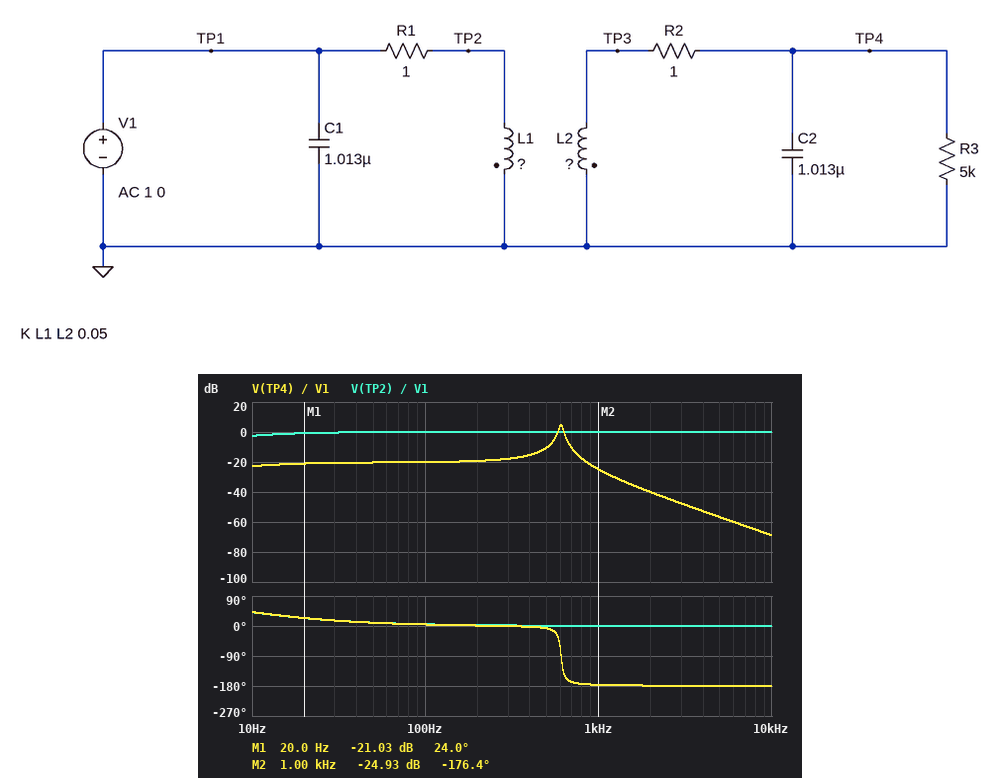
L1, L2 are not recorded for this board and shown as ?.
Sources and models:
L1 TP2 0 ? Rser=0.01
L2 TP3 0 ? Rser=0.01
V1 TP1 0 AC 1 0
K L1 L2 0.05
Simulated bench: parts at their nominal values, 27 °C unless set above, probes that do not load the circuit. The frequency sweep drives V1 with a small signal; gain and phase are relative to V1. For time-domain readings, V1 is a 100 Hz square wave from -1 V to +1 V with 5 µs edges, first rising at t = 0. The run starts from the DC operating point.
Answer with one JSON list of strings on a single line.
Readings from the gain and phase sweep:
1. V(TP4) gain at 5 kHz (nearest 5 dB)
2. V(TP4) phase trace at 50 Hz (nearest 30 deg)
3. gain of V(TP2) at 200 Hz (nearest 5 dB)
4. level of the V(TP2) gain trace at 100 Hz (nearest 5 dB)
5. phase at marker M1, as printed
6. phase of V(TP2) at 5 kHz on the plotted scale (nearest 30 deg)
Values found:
["-55 dB", "0 deg", "0 dB", "0 dB", "24.0 deg", "0 deg"]
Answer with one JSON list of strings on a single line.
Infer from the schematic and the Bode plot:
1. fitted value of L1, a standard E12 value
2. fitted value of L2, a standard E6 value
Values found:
["18 mH", "68 mH"]
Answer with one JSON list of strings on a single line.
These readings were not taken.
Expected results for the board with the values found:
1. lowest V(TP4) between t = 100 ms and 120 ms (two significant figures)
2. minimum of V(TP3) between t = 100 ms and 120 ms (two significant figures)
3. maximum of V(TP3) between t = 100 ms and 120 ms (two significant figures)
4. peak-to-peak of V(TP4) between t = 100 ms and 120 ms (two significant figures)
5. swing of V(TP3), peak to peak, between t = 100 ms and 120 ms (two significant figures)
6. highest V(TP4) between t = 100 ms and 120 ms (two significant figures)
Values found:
["-220 mV", "-220 mV", "220 mV", "440 mV", "440 mV", "220 mV"]
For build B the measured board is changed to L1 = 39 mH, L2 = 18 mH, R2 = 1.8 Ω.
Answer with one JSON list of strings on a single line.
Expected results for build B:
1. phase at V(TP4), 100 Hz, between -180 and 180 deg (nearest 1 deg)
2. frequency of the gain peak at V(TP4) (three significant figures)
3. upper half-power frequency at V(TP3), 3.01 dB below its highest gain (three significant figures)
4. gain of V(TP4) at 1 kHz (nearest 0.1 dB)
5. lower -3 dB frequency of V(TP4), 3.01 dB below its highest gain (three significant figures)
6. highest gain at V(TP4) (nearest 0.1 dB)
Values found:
["2 deg", "1.18 kHz", "1.20 kHz", "-18.5 dB", "1.16 kHz", "-1.5 dB"]
